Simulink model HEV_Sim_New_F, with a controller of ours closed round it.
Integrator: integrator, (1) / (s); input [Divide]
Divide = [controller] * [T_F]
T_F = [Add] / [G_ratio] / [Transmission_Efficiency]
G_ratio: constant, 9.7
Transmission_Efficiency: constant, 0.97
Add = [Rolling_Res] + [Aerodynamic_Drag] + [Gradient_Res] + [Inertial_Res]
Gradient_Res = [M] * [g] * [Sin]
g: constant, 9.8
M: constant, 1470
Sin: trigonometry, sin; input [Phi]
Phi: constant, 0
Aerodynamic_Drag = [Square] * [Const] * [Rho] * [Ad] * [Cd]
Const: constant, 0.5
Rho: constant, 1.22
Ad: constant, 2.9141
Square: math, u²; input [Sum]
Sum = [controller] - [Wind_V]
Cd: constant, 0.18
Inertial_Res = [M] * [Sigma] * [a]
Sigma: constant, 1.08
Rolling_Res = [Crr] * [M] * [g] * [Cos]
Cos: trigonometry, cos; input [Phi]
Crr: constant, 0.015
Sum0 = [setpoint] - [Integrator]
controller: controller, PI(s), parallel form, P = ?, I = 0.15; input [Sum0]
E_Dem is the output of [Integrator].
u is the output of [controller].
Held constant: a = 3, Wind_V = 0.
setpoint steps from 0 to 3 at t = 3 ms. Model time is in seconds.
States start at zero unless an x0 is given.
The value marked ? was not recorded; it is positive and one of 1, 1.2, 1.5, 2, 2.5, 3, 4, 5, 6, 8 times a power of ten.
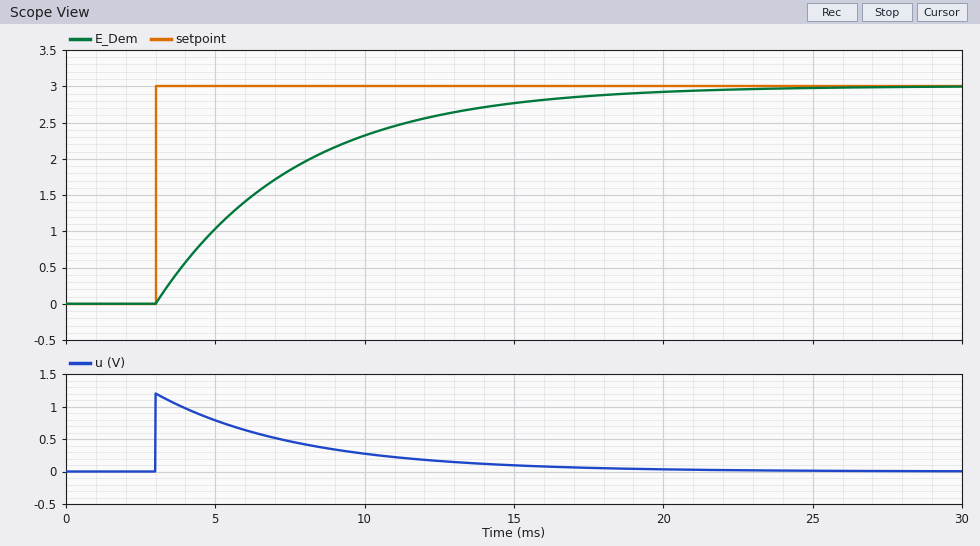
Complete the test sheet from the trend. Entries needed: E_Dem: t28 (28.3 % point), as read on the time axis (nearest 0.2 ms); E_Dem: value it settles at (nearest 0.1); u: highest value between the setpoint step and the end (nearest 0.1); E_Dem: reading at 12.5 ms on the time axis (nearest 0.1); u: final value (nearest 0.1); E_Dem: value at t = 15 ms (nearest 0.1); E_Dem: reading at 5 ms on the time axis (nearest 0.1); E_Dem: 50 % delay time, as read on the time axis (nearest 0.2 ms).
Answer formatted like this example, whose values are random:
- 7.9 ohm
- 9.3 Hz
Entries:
- 4.6 ms
- 3.0
- 1.2
- 2.6
- 0.0
- 2.8
- 1.0
- 6.2 ms
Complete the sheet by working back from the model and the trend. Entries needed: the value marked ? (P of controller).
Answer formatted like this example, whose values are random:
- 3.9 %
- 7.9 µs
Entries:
- 0.4
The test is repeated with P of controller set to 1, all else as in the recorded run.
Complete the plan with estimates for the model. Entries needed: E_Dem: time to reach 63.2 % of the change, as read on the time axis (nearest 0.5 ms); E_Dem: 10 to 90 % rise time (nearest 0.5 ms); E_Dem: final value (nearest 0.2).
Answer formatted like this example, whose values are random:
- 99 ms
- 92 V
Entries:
- 5.0 ms
- 4.0 ms
- 3.0
